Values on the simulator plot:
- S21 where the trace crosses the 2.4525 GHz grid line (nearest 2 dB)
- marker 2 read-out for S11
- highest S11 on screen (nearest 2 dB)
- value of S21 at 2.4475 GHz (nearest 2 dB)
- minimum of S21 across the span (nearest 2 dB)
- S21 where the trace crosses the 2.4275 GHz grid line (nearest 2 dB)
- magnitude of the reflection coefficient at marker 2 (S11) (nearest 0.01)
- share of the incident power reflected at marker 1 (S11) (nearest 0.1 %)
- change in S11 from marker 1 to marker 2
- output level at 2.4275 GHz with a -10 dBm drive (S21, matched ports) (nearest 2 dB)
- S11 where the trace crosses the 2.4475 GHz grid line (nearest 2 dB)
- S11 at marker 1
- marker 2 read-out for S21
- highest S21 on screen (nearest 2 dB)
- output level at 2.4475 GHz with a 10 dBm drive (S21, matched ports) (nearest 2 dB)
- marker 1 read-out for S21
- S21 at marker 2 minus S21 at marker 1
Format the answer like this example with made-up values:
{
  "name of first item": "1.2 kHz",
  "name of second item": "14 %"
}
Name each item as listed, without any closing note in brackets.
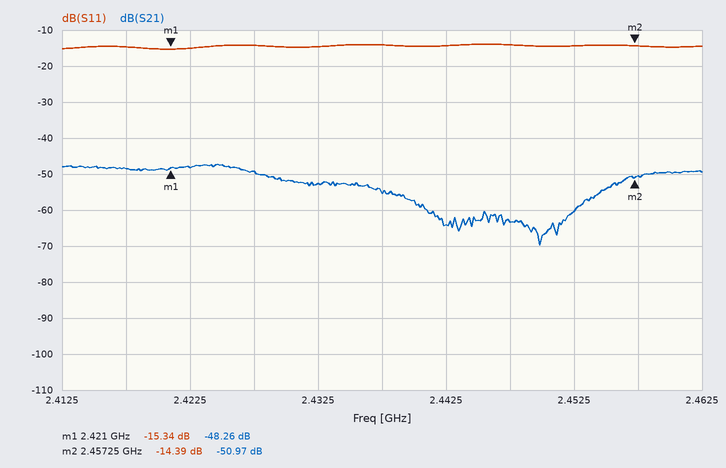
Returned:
{
  "S21 where the trace crosses the 2.4525 GHz grid line": "-60 dB",
  "marker 2 read-out for S11": "-14.39 dB",
  "highest S11 on screen": "-14 dB",
  "value of S21 at 2.4475 GHz": "-64 dB",
  "minimum of S21 across the span": "-70 dB",
  "S21 where the trace crosses the 2.4275 GHz grid line": "-50 dB",
  "magnitude of the reflection coefficient at marker 2 (S11)": "0.19",
  "share of the incident power reflected at marker 1 (S11)": "2.9 %",
  "change in S11 from marker 1 to marker 2": "0.95 dB",
  "output level at 2.4275 GHz with a -10 dBm drive (S21, matched ports)": "-60 dBm",
  "S11 where the trace crosses the 2.4475 GHz grid line": "-14 dB",
  "S11 at marker 1": "-15.34 dB",
  "marker 2 read-out for S21": "-50.97 dB",
  "highest S21 on screen": "-48 dB",
  "output level at 2.4475 GHz with a 10 dBm drive (S21, matched ports)": "-54 dBm",
  "marker 1 read-out for S21": "-48.26 dB",
  "S21 at marker 2 minus S21 at marker 1": "-2.71 dB"
}
